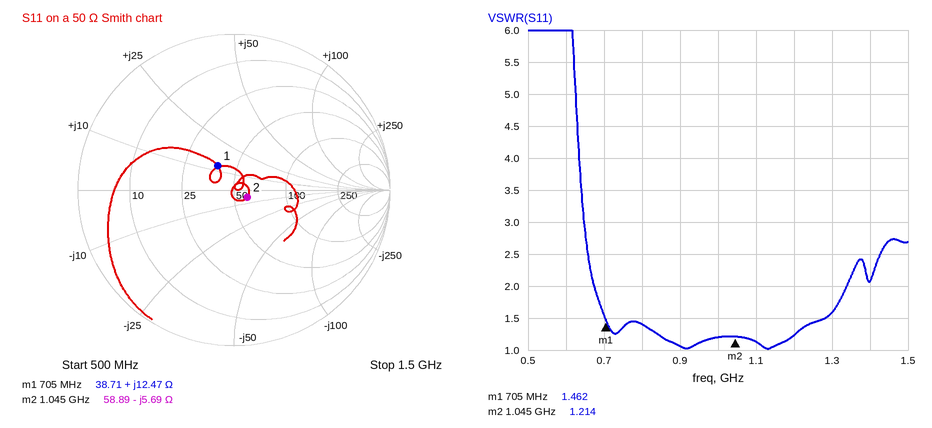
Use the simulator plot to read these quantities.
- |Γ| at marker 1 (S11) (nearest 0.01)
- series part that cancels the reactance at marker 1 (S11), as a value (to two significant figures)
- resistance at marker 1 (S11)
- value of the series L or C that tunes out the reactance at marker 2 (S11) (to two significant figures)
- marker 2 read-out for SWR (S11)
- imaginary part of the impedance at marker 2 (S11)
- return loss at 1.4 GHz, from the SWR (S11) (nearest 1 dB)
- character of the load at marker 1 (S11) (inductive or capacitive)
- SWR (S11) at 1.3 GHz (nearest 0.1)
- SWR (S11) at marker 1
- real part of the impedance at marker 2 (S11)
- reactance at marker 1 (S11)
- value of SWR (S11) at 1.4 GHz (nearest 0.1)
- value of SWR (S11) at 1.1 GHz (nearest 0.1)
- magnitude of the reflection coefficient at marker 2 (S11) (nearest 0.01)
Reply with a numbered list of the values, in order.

1. 0.19
2. 18 pF
3. 38.71 Ω
4. 870 pH
5. 1.214
6. -5.69 Ω
7. 9 dB
8. inductive
9. 1.6
10. 1.462
11. 58.89 Ω
12. +12.47 Ω
13. 2.1
14. 1.1
15. 0.10
